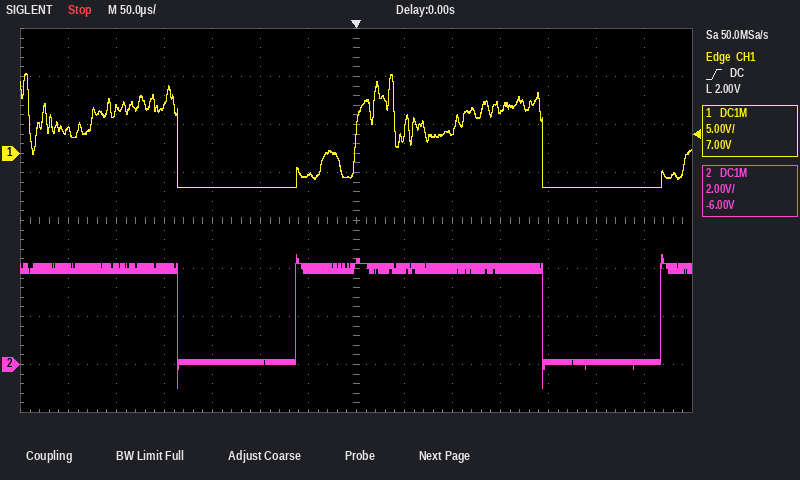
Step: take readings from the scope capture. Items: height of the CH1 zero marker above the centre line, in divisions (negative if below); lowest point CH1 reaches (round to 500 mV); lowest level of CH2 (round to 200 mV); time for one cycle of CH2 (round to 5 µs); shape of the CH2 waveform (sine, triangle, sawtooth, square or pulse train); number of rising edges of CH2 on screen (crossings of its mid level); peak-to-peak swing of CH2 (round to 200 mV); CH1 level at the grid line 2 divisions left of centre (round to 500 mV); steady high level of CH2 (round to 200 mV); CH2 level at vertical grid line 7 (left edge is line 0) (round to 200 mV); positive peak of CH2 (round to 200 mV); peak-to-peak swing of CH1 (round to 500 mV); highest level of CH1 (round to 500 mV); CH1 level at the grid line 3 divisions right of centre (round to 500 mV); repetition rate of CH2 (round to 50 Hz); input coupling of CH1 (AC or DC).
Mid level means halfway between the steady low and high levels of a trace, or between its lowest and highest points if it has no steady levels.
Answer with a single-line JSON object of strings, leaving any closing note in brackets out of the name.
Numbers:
{"height of the CH1 zero marker above the centre line, in divisions": "+1.4 div", "lowest point CH1 reaches": "-3.5 V", "lowest level of CH2": "-1.0 V", "time for one cycle of CH2": "380 µs", "shape of the CH2 waveform": "pulse train", "number of rising edges of CH2 on screen": "2", "peak-to-peak swing of CH2": "5.6 V", "CH1 level at the grid line 2 divisions left of centre": "-3.5 V", "steady high level of CH2": "4.0 V", "CH2 level at vertical grid line 7 (left edge is line 0)": "4.2 V", "positive peak of CH2": "4.6 V", "peak-to-peak swing of CH1": "12.0 V", "highest level of CH1": "8.5 V", "CH1 level at the grid line 3 divisions right of centre": "4.5 V", "repetition rate of CH2": "2.65 kHz", "input coupling of CH1": "DC"}
